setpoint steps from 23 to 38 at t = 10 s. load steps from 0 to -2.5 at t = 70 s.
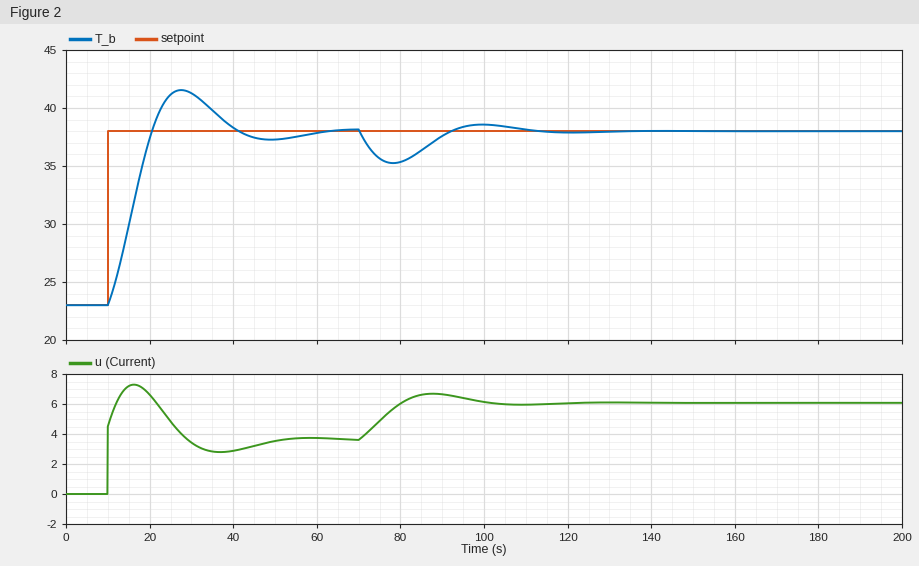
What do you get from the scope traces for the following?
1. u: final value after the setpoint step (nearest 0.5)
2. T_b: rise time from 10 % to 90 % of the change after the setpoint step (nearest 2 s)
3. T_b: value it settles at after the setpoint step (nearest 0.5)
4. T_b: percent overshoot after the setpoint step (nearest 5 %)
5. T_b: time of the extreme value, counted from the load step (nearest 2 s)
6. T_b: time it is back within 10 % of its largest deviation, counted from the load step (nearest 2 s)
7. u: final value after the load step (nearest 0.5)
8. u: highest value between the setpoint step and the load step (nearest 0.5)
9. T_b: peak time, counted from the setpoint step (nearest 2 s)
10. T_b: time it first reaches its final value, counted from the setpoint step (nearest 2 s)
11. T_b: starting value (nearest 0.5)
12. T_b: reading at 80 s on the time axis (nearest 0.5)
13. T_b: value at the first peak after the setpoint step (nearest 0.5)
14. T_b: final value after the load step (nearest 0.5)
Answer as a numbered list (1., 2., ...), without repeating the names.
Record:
1. 3.5
2. 8 s
3. 38.0
4. 25 %
5. 8 s
6. 38 s
7. 6.0
8. 7.5
9. 18 s
10. 10 s
11. 23.0
12. 35.5
13. 41.5
14. 38.0
